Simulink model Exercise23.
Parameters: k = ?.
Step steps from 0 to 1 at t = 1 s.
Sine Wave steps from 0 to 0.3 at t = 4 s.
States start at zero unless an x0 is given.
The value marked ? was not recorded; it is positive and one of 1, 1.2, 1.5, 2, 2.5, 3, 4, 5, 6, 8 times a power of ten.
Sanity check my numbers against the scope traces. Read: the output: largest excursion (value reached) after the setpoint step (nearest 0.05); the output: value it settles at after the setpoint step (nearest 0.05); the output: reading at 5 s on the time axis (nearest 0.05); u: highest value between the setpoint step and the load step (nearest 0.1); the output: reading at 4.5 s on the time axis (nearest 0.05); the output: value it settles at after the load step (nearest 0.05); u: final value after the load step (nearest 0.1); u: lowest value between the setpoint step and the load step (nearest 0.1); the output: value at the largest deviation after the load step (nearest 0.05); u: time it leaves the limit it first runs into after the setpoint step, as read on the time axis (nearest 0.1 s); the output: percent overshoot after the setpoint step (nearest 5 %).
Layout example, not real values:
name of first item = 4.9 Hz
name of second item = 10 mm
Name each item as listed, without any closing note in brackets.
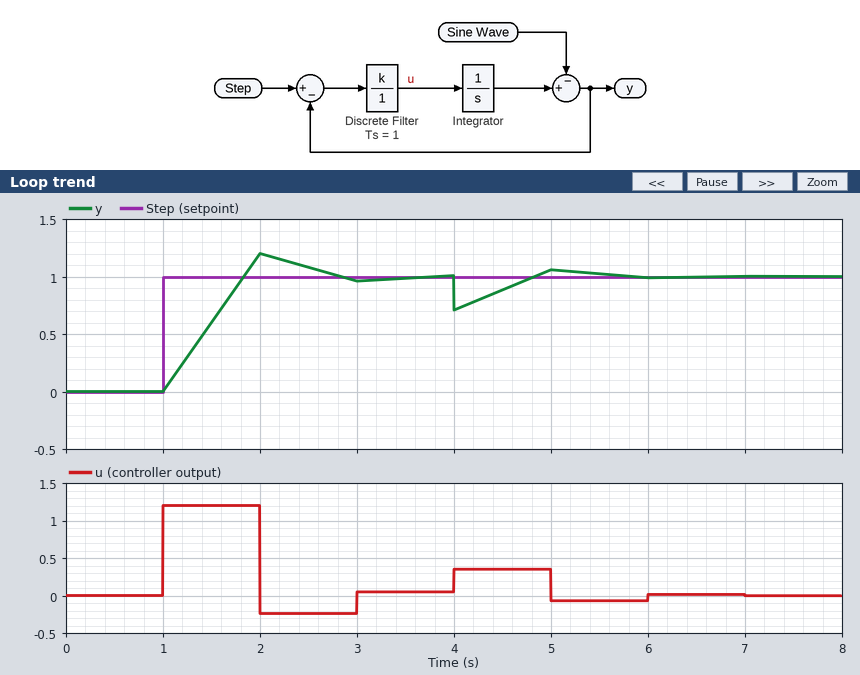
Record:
the output: largest excursion (value reached) after the setpoint step = 1.20
the output: value it settles at after the setpoint step = 1.00
the output: reading at 5 s on the time axis = 1.05
u: highest value between the setpoint step and the load step = 1.2
the output: reading at 4.5 s on the time axis = 0.90
the output: value it settles at after the load step = 1.00
u: final value after the load step = 0.0
u: lowest value between the setpoint step and the load step = -0.2
the output: value at the largest deviation after the load step = 0.70
u: time it leaves the limit it first runs into after the setpoint step, as read on the time axis = 2.0 s
the output: percent overshoot after the setpoint step = 20 %
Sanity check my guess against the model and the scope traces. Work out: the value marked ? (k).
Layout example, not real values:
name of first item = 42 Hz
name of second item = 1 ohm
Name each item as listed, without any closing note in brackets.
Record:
the value marked ? = 1.2
